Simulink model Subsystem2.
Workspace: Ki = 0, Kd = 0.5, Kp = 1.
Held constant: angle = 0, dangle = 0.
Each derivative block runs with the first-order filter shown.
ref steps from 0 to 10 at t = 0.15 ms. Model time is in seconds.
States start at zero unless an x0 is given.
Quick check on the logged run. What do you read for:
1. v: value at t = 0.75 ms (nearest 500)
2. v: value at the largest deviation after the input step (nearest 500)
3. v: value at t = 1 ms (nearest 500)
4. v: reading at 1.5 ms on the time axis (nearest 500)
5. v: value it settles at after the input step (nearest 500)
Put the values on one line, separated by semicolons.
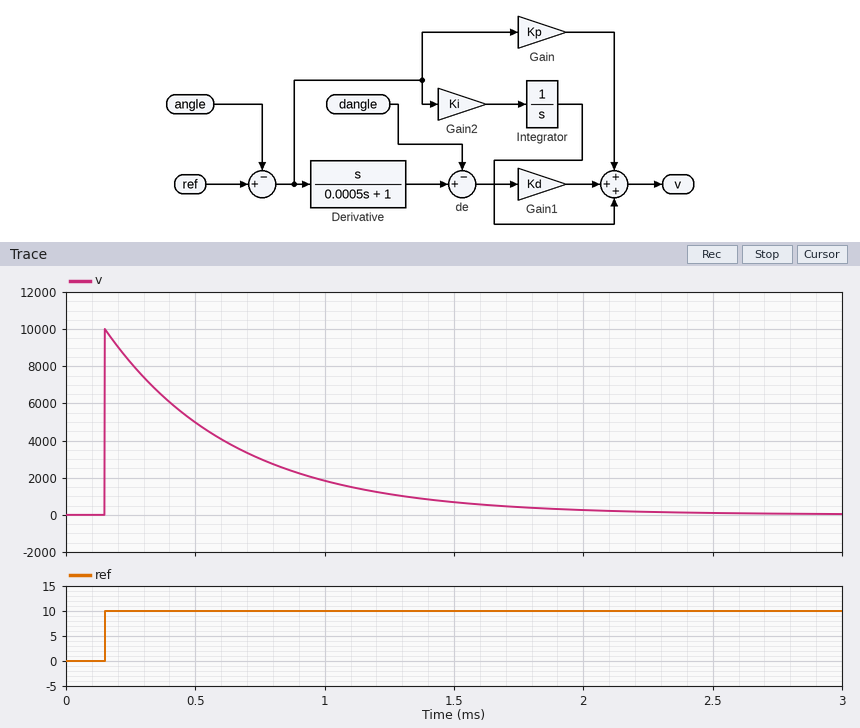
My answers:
3000; 10000; 2000; 500; 0
